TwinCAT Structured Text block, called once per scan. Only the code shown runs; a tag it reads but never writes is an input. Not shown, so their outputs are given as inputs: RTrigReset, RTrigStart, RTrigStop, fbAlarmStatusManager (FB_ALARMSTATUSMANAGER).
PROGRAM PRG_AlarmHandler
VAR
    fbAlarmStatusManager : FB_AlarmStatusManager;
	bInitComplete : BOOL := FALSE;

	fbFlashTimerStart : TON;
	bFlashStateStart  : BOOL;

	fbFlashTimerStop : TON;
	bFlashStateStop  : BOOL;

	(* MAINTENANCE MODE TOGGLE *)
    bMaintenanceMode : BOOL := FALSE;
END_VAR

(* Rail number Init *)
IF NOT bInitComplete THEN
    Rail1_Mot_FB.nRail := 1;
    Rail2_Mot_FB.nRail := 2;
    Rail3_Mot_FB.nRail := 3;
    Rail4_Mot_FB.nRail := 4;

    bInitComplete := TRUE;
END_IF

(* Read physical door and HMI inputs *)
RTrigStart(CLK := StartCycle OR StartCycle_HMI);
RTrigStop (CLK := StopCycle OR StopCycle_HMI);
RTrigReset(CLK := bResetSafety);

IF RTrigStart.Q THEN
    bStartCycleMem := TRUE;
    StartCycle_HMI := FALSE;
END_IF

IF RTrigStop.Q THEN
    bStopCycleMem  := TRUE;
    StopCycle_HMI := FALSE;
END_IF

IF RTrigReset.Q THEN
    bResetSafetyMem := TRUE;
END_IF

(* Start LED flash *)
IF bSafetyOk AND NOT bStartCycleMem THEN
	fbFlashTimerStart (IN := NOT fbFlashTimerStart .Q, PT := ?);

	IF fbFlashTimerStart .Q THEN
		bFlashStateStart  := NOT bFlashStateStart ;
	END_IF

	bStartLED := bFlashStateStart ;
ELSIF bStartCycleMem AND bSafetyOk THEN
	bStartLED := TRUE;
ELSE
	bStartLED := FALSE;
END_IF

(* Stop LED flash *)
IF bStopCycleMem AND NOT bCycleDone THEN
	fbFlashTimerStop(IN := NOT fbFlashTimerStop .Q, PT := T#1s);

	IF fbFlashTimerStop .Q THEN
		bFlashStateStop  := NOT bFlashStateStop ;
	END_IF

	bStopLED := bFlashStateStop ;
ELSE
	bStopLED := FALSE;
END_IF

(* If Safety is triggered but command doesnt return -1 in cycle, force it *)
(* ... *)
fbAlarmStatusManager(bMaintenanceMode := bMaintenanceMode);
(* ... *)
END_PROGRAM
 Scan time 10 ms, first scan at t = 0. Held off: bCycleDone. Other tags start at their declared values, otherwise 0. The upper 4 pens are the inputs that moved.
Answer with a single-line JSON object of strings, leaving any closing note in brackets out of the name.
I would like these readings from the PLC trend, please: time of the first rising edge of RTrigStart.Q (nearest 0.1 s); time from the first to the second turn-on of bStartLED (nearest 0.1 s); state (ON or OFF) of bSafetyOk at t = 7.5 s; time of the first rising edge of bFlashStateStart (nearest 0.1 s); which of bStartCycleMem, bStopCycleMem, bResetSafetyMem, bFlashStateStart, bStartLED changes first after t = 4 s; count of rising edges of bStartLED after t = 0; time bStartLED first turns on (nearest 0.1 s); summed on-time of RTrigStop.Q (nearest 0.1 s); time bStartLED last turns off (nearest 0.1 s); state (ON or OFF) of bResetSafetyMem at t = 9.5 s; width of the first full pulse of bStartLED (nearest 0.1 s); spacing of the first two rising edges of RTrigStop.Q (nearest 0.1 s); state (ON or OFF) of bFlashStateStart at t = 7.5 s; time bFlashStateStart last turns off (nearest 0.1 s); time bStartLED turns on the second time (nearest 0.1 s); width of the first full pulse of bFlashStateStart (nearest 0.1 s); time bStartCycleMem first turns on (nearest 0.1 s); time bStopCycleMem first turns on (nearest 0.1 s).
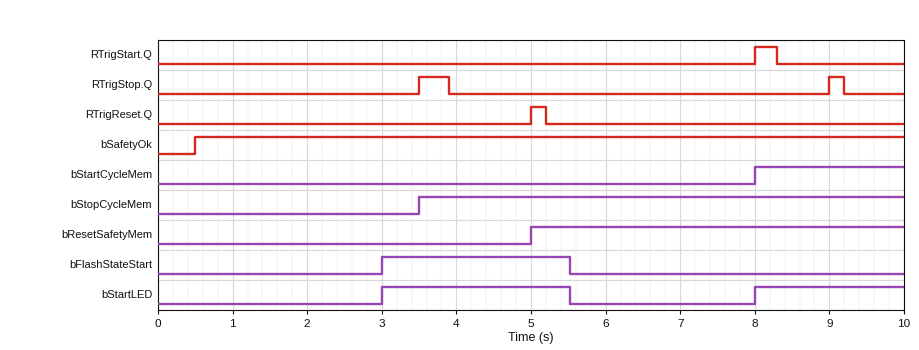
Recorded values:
{"time of the first rising edge of RTrigStart.Q": "8.0 s", "time from the first to the second turn-on of bStartLED": "5.0 s", "state (ON or OFF) of bSafetyOk at t = 7.5 s": "ON", "time of the first rising edge of bFlashStateStart": "3.0 s", "which of bStartCycleMem, bStopCycleMem, bResetSafetyMem, bFlashStateStart, bStartLED changes first after t = 4 s": "bResetSafetyMem", "count of rising edges of bStartLED after t = 0": "2", "time bStartLED first turns on": "3.0 s", "summed on-time of RTrigStop.Q": "0.6 s", "time bStartLED last turns off": "5.5 s", "state (ON or OFF) of bResetSafetyMem at t = 9.5 s": "ON", "width of the first full pulse of bStartLED": "2.5 s", "spacing of the first two rising edges of RTrigStop.Q": "5.5 s", "state (ON or OFF) of bFlashStateStart at t = 7.5 s": "OFF", "time bFlashStateStart last turns off": "5.5 s", "time bStartLED turns on the second time": "8.0 s", "width of the first full pulse of bFlashStateStart": "2.5 s", "time bStartCycleMem first turns on": "8.0 s", "time bStopCycleMem first turns on": "3.5 s"}
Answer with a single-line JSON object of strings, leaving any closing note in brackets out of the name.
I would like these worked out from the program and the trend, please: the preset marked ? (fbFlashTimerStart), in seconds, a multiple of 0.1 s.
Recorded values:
{"the preset marked ? (fbFlashTimerStart), in seconds, a multiple of 0.1 s": "2.5 s"}
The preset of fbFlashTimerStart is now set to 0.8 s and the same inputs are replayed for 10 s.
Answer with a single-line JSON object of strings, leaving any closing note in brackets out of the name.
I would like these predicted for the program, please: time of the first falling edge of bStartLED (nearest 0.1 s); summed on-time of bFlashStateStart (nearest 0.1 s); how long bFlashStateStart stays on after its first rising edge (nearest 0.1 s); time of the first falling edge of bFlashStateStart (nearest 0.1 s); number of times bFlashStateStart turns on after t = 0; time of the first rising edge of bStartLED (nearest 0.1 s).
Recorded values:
{"time of the first falling edge of bStartLED": "2.1 s", "summed on-time of bFlashStateStart": "5.4 s", "how long bFlashStateStart stays on after its first rising edge": "0.8 s", "time of the first falling edge of bFlashStateStart": "2.1 s", "number of times bFlashStateStart turns on after t = 0": "5", "time of the first rising edge of bStartLED": "1.3 s"}
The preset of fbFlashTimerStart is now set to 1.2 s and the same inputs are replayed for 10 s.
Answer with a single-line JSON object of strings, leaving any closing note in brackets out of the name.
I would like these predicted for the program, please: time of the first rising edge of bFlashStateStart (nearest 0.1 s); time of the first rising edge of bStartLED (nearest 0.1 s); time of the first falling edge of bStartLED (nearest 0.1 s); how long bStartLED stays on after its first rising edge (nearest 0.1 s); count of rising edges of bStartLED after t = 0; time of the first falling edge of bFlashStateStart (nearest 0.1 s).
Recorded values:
{"time of the first rising edge of bFlashStateStart": "1.7 s", "time of the first rising edge of bStartLED": "1.7 s", "time of the first falling edge of bStartLED": "2.9 s", "how long bStartLED stays on after its first rising edge": "1.2 s", "count of rising edges of bStartLED after t = 0": "4", "time of the first falling edge of bFlashStateStart": "2.9 s"}
